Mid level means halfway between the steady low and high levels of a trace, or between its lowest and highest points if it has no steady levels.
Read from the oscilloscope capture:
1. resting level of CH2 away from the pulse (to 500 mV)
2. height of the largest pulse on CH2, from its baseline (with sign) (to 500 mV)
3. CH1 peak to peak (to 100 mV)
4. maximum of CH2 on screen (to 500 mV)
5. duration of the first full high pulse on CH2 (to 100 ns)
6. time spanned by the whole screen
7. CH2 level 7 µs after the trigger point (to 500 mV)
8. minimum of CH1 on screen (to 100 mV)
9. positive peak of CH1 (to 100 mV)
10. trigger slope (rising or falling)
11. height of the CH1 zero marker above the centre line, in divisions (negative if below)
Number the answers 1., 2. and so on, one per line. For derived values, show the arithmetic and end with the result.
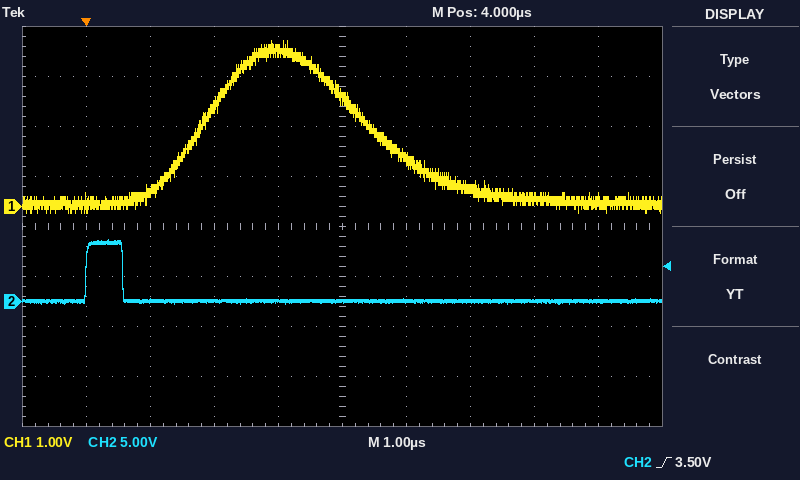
1. 0.0 V
2. 6.0 V − (0.0 V) = +6.0 V
3. 3.3 V − (-100 mV) = 3.4 V
4. 6.0 V
5. 600 ns
6. 10 µs
7. 0.0 V
8. -100 mV
9. 3.3 V
10. rising
11. +0.4 div
